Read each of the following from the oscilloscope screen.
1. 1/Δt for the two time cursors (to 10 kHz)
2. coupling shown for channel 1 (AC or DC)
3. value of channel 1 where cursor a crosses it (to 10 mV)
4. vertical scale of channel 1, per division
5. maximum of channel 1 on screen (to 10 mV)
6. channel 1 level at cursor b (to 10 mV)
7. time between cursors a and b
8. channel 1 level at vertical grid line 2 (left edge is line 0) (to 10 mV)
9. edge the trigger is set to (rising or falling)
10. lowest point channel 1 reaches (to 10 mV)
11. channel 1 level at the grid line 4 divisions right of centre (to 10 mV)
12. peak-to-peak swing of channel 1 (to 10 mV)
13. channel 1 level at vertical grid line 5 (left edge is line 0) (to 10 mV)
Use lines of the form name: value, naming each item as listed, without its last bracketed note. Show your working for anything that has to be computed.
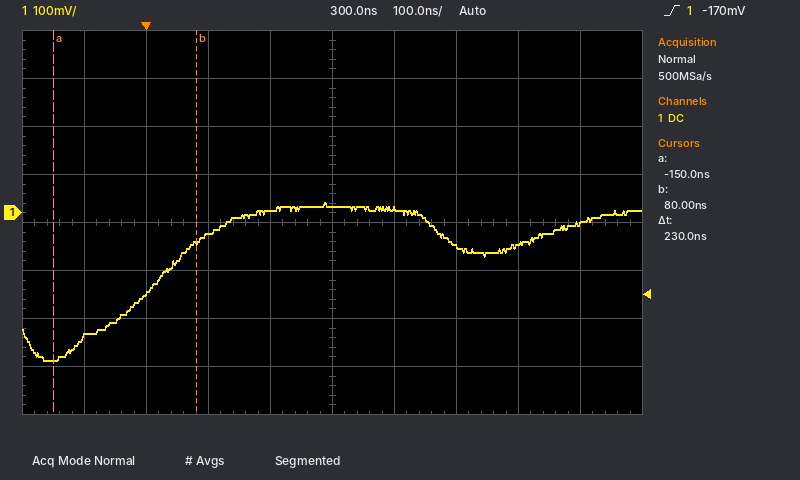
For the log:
1/Δt for the two time cursors: 1 / 230 ns ≈ 4.35 MHz
coupling shown for channel 1: DC
value of channel 1 where cursor a crosses it: -310 mV
vertical scale of channel 1, per division: 100 mV
maximum of channel 1 on screen: 20 mV
channel 1 level at cursor b: -60 mV
time between cursors a and b: 230 ns
channel 1 level at vertical grid line 2 (left edge is line 0): -170 mV
edge the trigger is set to: rising
lowest point channel 1 reaches: -310 mV
channel 1 level at the grid line 4 divisions right of centre: -20 mV
peak-to-peak swing of channel 1: 20 mV − (-310 mV) = 330 mV
channel 1 level at vertical grid line 5 (left edge is line 0): 10 mV
